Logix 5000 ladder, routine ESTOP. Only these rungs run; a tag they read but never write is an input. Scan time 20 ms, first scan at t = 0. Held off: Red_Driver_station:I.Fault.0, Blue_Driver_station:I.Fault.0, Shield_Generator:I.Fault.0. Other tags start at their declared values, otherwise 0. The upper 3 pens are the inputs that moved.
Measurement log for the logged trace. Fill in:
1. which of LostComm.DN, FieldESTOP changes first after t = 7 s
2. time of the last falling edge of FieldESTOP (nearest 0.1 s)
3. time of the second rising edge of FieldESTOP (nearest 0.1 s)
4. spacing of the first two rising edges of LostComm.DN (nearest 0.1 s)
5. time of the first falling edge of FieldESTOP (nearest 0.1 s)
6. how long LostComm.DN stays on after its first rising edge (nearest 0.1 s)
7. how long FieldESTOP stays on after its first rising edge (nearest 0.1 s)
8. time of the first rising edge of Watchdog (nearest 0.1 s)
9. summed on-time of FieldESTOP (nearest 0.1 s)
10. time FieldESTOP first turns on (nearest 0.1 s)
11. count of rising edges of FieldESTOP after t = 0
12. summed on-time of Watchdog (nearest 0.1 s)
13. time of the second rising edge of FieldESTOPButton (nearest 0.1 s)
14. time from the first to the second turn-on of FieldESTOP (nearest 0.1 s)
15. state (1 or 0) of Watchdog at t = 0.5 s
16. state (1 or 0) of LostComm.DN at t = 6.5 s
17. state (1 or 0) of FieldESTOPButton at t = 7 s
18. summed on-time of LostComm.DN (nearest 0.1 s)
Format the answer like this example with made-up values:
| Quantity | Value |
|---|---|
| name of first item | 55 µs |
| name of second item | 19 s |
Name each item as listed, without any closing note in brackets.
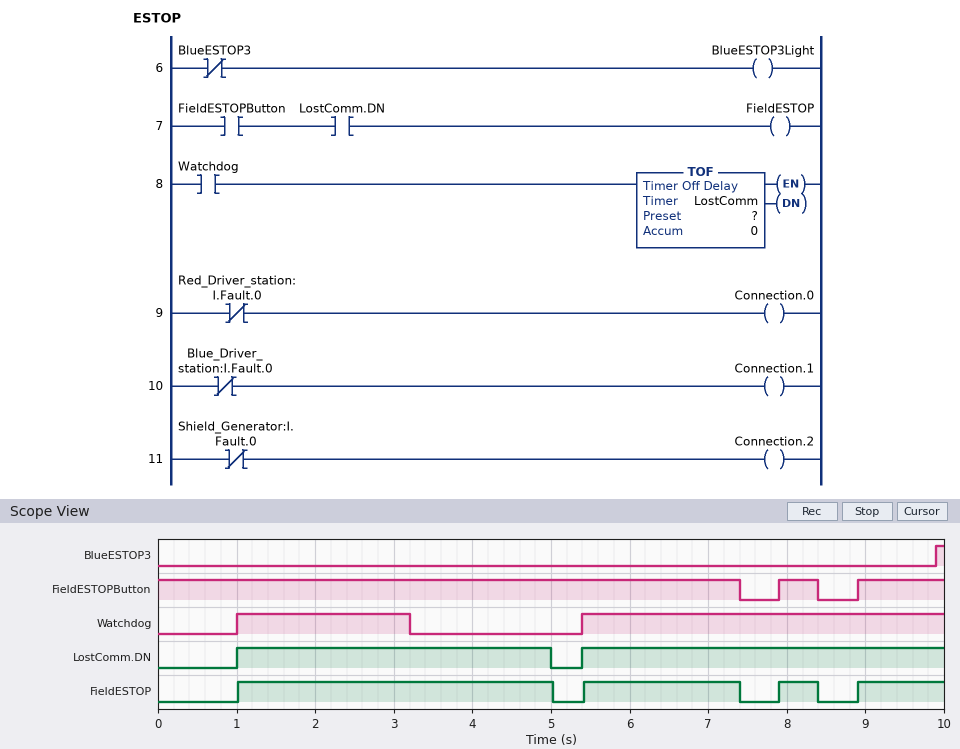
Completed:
| Quantity | Value |
|---|---|
| which of LostComm.DN, FieldESTOP changes first after t = 7 s | FieldESTOP |
| time of the last falling edge of FieldESTOP | 8.4 s |
| time of the second rising edge of FieldESTOP | 5.4 s |
| spacing of the first two rising edges of LostComm.DN | 4.4 s |
| time of the first falling edge of FieldESTOP | 5.0 s |
| how long LostComm.DN stays on after its first rising edge | 4.0 s |
| how long FieldESTOP stays on after its first rising edge | 4.0 s |
| time of the first rising edge of Watchdog | 1.0 s |
| summed on-time of FieldESTOP | 7.6 s |
| time FieldESTOP first turns on | 1.0 s |
| count of rising edges of FieldESTOP after t = 0 | 4 |
| summed on-time of Watchdog | 6.8 s |
| time of the second rising edge of FieldESTOPButton | 8.9 s |
| time from the first to the second turn-on of FieldESTOP | 4.4 s |
| state (1 or 0) of Watchdog at t = 0.5 s | 0 |
| state (1 or 0) of LostComm.DN at t = 6.5 s | 1 |
| state (1 or 0) of FieldESTOPButton at t = 7 s | 1 |
| summed on-time of LostComm.DN | 8.6 s |
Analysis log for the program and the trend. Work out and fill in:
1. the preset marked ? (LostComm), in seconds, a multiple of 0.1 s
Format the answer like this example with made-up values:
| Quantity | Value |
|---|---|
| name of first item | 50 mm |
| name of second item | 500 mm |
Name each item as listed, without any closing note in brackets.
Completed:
| Quantity | Value |
|---|---|
| the preset marked ? (LostComm), in seconds, a multiple of 0.1 s | 1.8 s |
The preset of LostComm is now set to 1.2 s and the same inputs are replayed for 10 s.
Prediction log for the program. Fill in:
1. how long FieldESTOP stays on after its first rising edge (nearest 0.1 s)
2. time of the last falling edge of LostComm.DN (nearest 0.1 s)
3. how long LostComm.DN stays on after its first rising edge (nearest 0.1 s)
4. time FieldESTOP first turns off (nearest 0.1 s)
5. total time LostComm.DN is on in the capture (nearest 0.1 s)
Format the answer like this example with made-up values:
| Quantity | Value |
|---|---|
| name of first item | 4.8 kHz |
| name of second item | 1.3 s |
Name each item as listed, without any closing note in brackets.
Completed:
| Quantity | Value |
|---|---|
| how long FieldESTOP stays on after its first rising edge | 3.4 s |
| time of the last falling edge of LostComm.DN | 4.4 s |
| how long LostComm.DN stays on after its first rising edge | 3.4 s |
| time FieldESTOP first turns off | 4.4 s |
| total time LostComm.DN is on in the capture | 8.0 s |
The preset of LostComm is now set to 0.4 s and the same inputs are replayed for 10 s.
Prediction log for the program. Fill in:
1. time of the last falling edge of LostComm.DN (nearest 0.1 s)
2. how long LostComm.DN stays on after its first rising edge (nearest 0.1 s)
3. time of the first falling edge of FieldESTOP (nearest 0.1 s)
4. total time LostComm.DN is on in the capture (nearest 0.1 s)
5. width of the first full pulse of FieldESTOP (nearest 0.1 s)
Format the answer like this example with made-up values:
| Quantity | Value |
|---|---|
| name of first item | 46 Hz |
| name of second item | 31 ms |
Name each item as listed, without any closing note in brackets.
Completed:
| Quantity | Value |
|---|---|
| time of the last falling edge of LostComm.DN | 3.6 s |
| how long LostComm.DN stays on after its first rising edge | 2.6 s |
| time of the first falling edge of FieldESTOP | 3.6 s |
| total time LostComm.DN is on in the capture | 7.2 s |
| width of the first full pulse of FieldESTOP | 2.6 s |
